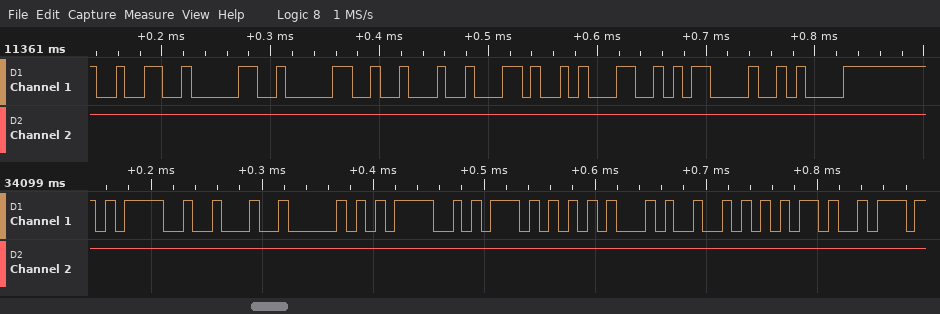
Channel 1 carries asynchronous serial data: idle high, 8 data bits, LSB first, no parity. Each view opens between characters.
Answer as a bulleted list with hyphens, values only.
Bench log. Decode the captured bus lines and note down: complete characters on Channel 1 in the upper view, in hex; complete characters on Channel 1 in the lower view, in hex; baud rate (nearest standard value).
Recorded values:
- 32, 30, 30, 22, 2C, 31, 0D, 0A
- 3D, 22, 50, 4F, 57, 45, 52, 2D
- 115200 baud
